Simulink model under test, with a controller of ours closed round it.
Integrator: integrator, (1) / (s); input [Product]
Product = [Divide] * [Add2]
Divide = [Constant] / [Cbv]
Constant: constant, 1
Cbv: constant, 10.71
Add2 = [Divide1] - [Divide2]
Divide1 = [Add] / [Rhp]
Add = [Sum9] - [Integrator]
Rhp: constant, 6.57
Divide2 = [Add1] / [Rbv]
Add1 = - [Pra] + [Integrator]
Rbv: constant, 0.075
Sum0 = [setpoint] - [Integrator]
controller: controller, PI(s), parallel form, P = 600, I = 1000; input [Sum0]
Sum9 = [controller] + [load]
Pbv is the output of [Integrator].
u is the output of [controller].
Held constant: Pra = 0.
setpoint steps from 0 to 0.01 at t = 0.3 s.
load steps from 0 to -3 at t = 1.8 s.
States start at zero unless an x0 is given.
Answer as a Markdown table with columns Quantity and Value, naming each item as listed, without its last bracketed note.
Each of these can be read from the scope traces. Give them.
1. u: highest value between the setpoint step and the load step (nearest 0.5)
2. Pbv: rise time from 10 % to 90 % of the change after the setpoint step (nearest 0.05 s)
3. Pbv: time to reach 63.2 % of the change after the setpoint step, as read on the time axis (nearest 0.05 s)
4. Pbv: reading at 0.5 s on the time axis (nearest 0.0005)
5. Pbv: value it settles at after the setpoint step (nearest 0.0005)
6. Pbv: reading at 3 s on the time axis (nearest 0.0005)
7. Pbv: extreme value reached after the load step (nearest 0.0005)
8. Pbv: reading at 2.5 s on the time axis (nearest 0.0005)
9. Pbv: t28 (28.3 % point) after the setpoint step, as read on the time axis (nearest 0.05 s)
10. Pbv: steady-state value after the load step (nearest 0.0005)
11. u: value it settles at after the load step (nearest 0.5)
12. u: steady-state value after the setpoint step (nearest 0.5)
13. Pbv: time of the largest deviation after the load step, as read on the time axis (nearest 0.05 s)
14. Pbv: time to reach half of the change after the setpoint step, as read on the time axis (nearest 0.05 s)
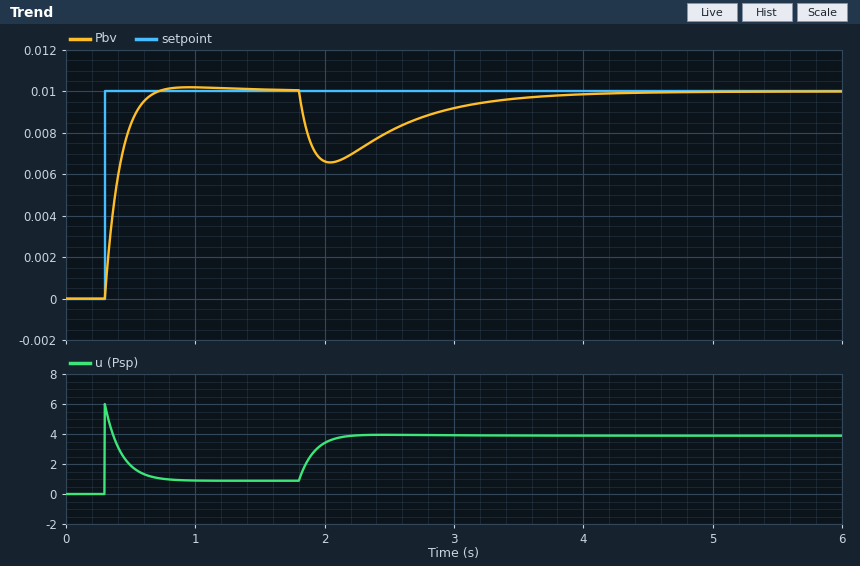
| Quantity | Value |
|---|---|
| u: highest value between the setpoint step and the load step | 6.0 |
| Pbv: rise time from 10 % to 90 % of the change after the setpoint step | 0.25 s |
| Pbv: time to reach 63.2 % of the change after the setpoint step, as read on the time axis | 0.40 s |
| Pbv: reading at 0.5 s on the time axis | 0.0085 |
| Pbv: value it settles at after the setpoint step | 0.0100 |
| Pbv: reading at 3 s on the time axis | 0.0090 |
| Pbv: extreme value reached after the load step | 0.0065 |
| Pbv: reading at 2.5 s on the time axis | 0.0080 |
| Pbv: t28 (28.3 % point) after the setpoint step, as read on the time axis | 0.35 s |
| Pbv: steady-state value after the load step | 0.0100 |
| u: value it settles at after the load step | 4.0 |
| u: steady-state value after the setpoint step | 1.0 |
| Pbv: time of the largest deviation after the load step, as read on the time axis | 2.05 s |
| Pbv: time to reach half of the change after the setpoint step, as read on the time axis | 0.40 s |
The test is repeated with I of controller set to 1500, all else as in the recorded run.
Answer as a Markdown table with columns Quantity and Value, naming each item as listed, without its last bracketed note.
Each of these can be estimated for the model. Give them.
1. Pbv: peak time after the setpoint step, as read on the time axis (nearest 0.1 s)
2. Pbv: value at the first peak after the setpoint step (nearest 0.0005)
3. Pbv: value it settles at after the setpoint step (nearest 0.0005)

| Quantity | Value |
|---|---|
| Pbv: peak time after the setpoint step, as read on the time axis | 0.8 s |
| Pbv: value at the first peak after the setpoint step | 0.0105 |
| Pbv: value it settles at after the setpoint step | 0.0100 |
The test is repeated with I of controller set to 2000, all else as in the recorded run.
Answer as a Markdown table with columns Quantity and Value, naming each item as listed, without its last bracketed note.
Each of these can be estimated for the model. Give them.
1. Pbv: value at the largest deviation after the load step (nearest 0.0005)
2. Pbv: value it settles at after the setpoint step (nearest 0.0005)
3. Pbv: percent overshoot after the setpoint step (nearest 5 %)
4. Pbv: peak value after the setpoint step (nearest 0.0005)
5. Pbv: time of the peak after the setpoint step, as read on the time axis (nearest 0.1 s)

| Quantity | Value |
|---|---|
| Pbv: value at the largest deviation after the load step | 0.0070 |
| Pbv: value it settles at after the setpoint step | 0.0100 |
| Pbv: percent overshoot after the setpoint step | 10 % |
| Pbv: peak value after the setpoint step | 0.0110 |
| Pbv: time of the peak after the setpoint step, as read on the time axis | 0.7 s |
